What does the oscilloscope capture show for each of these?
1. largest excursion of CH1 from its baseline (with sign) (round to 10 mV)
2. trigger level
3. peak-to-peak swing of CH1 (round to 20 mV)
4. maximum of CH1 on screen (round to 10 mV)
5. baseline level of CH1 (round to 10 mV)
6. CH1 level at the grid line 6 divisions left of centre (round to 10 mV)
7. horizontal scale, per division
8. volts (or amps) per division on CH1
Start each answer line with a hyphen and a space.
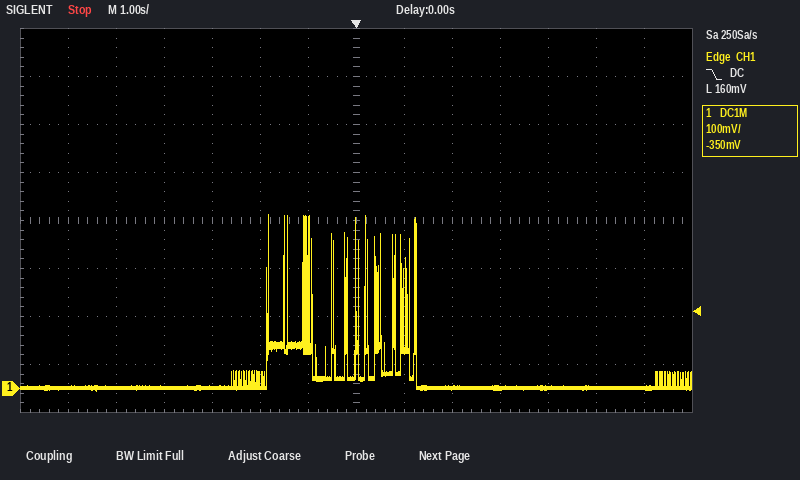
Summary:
- +360 mV
- 160 mV
- 360 mV
- 360 mV
- 0 mV
- 0 mV
- 1 s
- 100 mV
